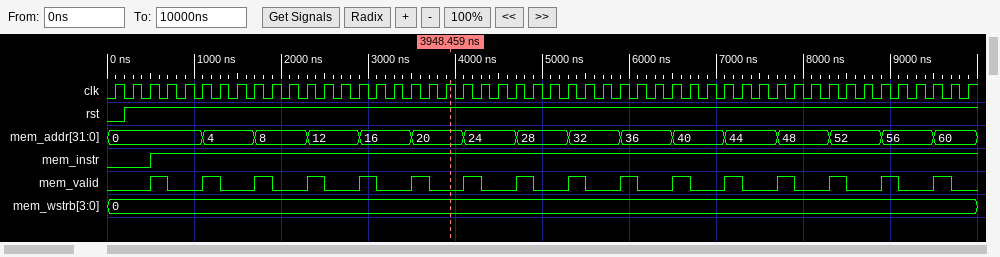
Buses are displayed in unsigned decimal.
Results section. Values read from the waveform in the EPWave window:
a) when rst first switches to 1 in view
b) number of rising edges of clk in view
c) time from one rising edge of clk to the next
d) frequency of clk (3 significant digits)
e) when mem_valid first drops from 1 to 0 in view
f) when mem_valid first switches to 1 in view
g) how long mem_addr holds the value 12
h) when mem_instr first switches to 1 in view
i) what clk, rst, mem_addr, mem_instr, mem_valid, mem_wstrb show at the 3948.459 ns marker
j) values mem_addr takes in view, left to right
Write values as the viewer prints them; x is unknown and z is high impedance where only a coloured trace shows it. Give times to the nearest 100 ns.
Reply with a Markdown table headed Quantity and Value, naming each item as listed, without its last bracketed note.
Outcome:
| Quantity | Value |
|---|---|
| when rst first switches to 1 in view | 200 ns |
| number of rising edges of clk in view | 50 |
| time from one rising edge of clk to the next | 200 ns |
| frequency of clk | 5.00 MHz |
| when mem_valid first drops from 1 to 0 in view | 700 ns |
| when mem_valid first switches to 1 in view | 500 ns |
| how long mem_addr holds the value 12 | 600 ns |
| when mem_instr first switches to 1 in view | 500 ns |
| what clk, rst, mem_addr, mem_instr, mem_valid, mem_wstrb show at the 3948.459 ns marker | clk=1, rst=1, mem_addr=20, mem_instr=1, mem_valid=0, mem_wstrb=0 |
| values mem_addr takes in view, left to right | 0, 4, 8, 12, 16, 20, 24, 28, 32, 36, 40, 44, 48, 52, 56, 60 |
